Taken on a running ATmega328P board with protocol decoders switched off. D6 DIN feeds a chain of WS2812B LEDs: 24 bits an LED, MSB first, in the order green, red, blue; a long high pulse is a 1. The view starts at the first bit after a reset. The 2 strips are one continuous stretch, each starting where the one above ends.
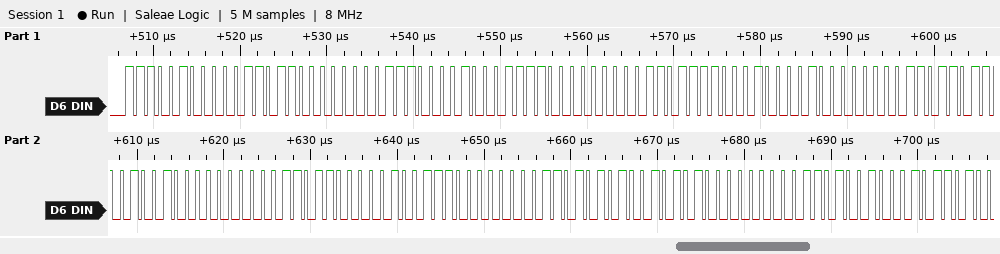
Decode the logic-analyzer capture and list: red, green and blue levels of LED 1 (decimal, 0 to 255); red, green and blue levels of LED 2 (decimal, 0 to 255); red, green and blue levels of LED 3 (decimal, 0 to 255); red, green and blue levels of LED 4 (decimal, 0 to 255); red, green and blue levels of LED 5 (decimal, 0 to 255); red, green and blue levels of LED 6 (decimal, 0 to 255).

27, 228, 0
30, 225, 0
33, 222, 0
36, 219, 0
39, 216, 0
42, 213, 0
